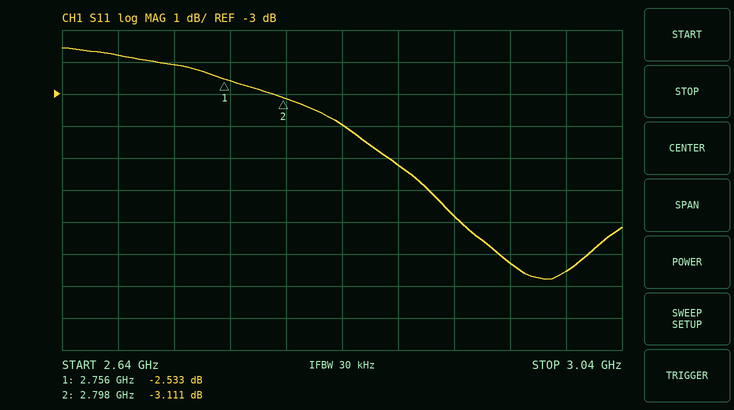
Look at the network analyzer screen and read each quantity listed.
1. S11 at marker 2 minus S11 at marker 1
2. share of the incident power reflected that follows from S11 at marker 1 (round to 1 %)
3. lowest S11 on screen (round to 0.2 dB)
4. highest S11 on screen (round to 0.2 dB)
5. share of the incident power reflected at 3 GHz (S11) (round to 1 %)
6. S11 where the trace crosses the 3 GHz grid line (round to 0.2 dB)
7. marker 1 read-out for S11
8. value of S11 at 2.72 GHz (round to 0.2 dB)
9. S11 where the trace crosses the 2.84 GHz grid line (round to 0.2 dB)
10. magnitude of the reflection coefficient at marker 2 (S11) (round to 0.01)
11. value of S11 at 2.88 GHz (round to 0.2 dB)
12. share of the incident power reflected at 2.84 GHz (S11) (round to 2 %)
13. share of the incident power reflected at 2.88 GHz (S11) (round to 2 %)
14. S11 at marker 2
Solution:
-0.578 dB
56 %
-8.8 dB
-1.6 dB
14 %
-8.6 dB
-2.533 dB
-2.0 dB
-4.0 dB
0.70
-5.2 dB
40 %
30 %
-3.111 dB
